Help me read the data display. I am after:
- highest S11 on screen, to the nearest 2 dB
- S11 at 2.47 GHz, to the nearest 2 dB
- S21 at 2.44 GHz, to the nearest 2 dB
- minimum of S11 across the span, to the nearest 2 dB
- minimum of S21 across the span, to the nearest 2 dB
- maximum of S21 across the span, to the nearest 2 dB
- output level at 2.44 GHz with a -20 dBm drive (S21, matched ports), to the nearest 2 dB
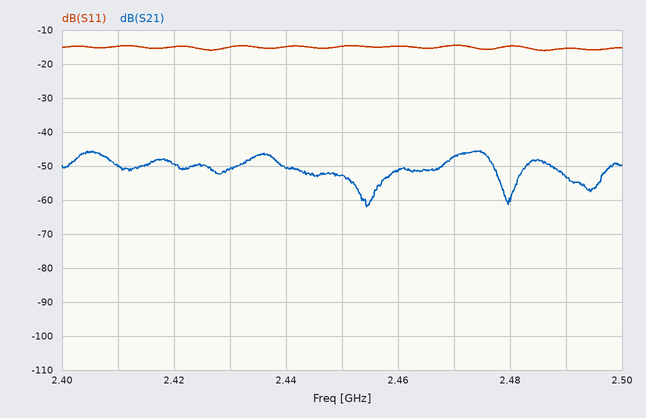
-14 dB
-14 dB
-50 dB
-16 dB
-62 dB
-46 dB
-70 dBm
